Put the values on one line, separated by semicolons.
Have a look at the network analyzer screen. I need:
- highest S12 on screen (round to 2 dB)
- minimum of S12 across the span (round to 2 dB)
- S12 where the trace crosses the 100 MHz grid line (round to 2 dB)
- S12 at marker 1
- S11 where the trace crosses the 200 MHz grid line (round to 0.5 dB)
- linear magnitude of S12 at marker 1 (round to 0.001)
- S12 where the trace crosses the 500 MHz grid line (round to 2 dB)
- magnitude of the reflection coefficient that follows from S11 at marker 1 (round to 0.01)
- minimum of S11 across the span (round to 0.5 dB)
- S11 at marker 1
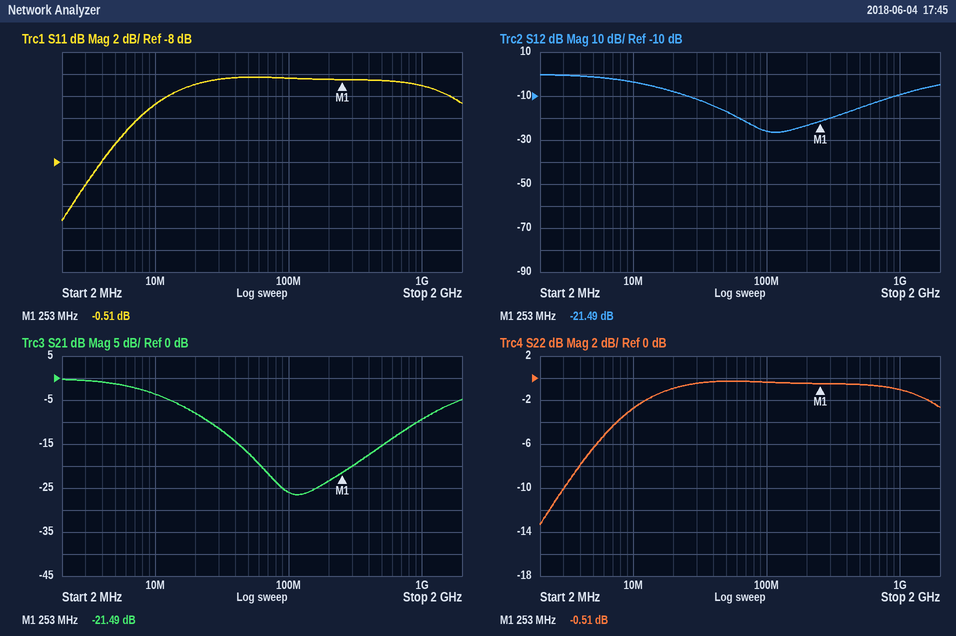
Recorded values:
0 dB; -26 dB; -26 dB; -21.49 dB; -0.5 dB; 0.084; -16 dB; 0.94; -13.5 dB; -0.51 dB
